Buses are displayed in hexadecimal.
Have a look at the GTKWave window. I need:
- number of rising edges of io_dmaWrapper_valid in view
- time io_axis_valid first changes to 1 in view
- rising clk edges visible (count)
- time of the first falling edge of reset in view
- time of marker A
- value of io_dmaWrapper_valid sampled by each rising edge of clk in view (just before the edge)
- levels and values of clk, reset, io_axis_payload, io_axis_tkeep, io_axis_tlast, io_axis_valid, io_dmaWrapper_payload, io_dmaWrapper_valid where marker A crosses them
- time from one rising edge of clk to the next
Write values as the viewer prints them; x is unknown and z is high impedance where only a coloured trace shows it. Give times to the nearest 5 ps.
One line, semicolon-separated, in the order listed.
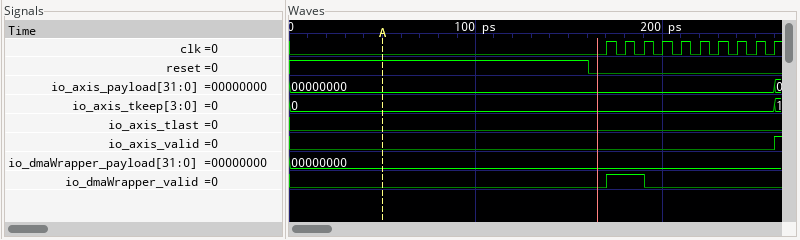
1; 260 ps; 10; 160 ps; 50 ps; 0 1 1 0 0 0 0 0 0 0; clk=0, reset=1, io_axis_payload=00000000, io_axis_tkeep=0, io_axis_tlast=0, io_axis_valid=0, io_dmaWrapper_payload=00000000, io_dmaWrapper_valid=0; 10 ps
